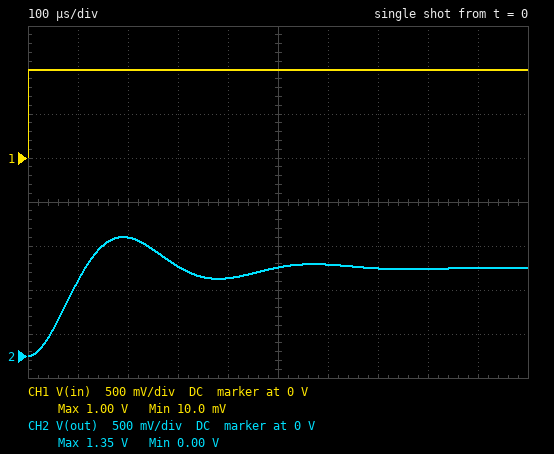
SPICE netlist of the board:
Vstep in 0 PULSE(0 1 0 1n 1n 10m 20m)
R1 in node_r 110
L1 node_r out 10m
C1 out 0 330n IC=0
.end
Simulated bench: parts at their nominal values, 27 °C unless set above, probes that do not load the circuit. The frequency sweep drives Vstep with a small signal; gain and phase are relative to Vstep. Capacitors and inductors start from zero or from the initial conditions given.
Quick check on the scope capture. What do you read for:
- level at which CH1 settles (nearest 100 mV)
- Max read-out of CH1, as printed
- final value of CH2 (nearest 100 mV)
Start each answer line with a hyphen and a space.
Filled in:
- 1.0 V
- 1.00 V
- 1.0 V
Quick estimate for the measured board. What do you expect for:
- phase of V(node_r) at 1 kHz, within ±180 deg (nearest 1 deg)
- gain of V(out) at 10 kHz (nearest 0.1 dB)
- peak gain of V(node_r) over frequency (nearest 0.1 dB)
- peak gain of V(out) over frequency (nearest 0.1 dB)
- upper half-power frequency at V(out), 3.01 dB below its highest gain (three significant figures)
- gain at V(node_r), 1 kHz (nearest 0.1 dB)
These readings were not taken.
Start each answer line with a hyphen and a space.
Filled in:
- -15 deg
- -21.8 dB
- 0 dB
- 4.4 dB
- 3.28 kHz
- -0.3 dB
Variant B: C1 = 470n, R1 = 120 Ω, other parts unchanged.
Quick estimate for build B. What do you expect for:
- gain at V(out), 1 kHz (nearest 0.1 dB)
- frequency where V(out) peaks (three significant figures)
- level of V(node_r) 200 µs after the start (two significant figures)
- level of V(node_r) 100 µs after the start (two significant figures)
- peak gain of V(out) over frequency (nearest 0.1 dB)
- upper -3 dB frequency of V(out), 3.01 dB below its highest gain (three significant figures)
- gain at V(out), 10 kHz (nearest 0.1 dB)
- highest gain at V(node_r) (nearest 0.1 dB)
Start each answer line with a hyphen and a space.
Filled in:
- 1.0 dB
- 1.89 kHz
- 870 mV
- 520 mV
- 2.5 dB
- 2.76 kHz
- -25.1 dB
- 0 dB
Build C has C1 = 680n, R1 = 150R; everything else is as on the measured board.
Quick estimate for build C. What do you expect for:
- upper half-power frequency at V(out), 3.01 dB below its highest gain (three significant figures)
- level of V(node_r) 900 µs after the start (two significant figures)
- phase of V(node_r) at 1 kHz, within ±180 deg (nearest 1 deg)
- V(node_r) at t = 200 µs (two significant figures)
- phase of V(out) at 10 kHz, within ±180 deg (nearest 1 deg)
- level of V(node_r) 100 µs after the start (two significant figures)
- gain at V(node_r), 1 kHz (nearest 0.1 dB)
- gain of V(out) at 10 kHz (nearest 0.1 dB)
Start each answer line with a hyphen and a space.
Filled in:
- 2.12 kHz
- 1.0 V
- -41 deg
- 670 mV
- -166 deg
- 390 mV
- -2.5 dB
- -28.5 dB
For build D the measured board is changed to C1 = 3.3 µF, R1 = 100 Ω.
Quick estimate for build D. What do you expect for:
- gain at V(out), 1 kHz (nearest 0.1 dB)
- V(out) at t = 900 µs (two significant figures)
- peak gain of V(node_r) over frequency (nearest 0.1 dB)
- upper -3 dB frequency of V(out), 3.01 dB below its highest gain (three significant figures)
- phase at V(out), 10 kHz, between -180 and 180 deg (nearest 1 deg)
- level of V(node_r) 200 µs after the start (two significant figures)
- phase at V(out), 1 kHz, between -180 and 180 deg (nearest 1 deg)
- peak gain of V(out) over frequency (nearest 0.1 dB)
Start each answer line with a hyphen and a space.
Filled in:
- -6.4 dB
- 980 mV
- 0 dB
- 645 Hz
- -171 deg
- 290 mV
- -98 deg
- 0 dB
